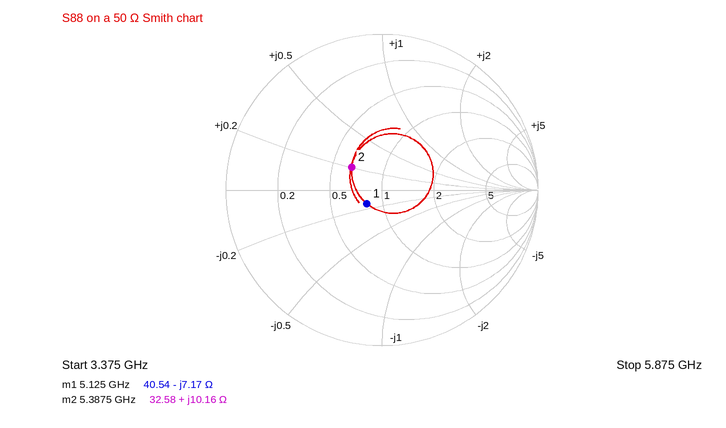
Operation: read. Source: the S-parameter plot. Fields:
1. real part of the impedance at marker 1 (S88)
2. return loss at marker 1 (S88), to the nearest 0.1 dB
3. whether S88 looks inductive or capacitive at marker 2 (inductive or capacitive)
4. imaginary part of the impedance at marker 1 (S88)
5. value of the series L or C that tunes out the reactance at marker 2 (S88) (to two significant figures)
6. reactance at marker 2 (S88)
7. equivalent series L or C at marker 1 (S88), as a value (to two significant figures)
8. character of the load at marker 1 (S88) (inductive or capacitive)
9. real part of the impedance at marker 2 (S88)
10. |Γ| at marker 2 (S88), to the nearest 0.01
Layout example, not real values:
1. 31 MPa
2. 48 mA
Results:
1. 40.54 Ω
2. 17.7 dB
3. inductive
4. -7.17 Ω
5. 2.9 pF
6. +10.16 Ω
7. 4.3 pF
8. capacitive
9. 32.58 Ω
10. 0.24
